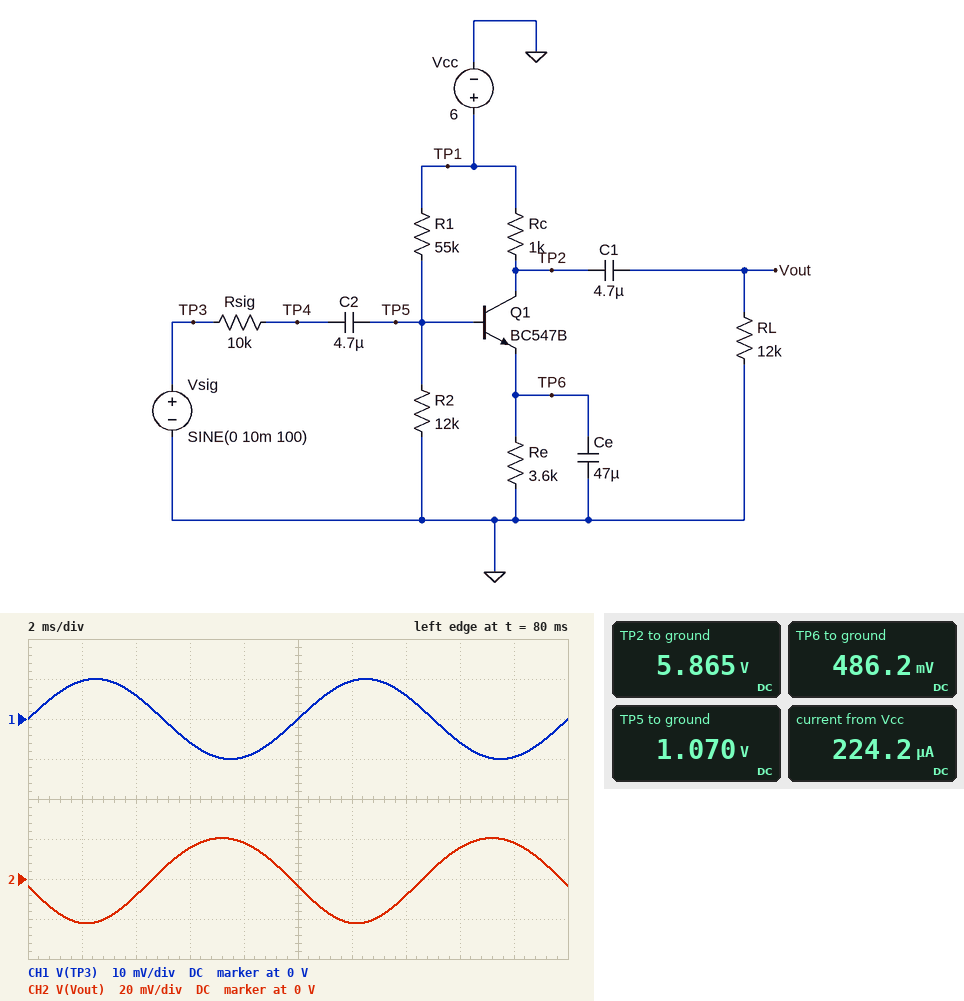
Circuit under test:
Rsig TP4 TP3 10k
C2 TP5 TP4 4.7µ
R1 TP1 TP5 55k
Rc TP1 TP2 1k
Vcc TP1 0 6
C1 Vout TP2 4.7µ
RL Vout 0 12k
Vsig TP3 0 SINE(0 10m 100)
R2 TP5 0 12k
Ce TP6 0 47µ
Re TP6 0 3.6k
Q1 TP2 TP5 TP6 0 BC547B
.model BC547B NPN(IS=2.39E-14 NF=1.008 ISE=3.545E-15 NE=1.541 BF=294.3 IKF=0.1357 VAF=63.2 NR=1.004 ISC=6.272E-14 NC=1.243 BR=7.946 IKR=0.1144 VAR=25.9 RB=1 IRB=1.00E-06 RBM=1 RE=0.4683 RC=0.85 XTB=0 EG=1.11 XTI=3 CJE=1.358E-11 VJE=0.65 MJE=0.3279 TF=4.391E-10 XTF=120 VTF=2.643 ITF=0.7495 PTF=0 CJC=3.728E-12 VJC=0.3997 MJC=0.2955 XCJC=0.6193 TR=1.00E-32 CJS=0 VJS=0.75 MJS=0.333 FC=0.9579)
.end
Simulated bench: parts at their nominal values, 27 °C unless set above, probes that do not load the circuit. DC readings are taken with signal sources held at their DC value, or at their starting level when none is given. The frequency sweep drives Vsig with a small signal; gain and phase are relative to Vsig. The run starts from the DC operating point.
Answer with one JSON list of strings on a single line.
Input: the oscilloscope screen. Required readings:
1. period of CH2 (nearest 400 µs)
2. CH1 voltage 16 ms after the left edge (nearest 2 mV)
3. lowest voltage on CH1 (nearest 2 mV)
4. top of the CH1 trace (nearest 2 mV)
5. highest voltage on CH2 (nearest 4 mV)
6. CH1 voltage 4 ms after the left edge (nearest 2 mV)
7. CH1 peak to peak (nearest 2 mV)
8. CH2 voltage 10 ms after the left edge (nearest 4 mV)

["10.0 ms", "-6 mV", "-10 mV", "10 mV", "20 mV", "6 mV", "20 mV", "-4 mV"]
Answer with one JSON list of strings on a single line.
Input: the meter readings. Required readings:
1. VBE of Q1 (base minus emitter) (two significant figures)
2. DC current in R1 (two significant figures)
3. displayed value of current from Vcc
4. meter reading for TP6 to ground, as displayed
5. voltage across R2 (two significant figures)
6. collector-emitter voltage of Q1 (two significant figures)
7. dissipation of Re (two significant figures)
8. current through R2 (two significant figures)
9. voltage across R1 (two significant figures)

["580 mV", "90 µA", "224.2 µA", "486.2 mV", "1.1 V", "5.4 V", "66 µW", "89 µA", "4.9 V"]
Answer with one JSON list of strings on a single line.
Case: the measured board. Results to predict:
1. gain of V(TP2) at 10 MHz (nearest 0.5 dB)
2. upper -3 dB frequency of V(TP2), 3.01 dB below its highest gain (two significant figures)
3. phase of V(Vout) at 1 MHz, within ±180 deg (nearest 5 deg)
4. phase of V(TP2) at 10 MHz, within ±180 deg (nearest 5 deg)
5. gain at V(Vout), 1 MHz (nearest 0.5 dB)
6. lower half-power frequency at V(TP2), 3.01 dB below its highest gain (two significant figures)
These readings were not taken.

["-15.0 dB", "850 kHz", "130 deg", "90 deg", "3.0 dB", "17 Hz"]
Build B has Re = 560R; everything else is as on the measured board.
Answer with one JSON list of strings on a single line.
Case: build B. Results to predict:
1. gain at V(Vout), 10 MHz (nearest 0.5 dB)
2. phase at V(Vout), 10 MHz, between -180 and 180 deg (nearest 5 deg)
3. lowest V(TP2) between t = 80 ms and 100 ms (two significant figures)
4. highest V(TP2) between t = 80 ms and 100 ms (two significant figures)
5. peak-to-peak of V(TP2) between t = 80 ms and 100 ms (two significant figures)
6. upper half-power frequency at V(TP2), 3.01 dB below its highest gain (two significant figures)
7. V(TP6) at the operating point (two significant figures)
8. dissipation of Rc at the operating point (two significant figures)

["-8.0 dB", "90 deg", "5.2 V", "5.3 V", "140 mV", "460 kHz", "420 mV", "560 µW"]
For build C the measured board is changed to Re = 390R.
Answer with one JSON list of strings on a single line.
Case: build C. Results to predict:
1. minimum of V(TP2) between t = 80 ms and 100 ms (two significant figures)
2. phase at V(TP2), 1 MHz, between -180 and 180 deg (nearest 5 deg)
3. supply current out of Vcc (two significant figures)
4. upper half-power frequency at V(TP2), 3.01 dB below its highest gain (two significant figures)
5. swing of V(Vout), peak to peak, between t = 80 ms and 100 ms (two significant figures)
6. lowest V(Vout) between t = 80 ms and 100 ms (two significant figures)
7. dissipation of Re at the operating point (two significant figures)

["4.9 V", "110 deg", "1.1 mA", "410 kHz", "160 mV", "-81 mV", "420 µW"]
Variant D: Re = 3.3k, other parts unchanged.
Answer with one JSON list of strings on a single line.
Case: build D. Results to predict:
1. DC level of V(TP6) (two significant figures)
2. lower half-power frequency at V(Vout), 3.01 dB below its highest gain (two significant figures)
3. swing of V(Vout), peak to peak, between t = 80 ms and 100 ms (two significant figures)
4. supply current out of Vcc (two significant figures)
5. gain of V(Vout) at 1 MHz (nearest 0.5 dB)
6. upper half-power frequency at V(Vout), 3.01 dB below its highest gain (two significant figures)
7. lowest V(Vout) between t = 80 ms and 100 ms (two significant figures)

["480 mV", "19 Hz", "46 mV", "240 µA", "3.5 dB", "830 kHz", "-24 mV"]
